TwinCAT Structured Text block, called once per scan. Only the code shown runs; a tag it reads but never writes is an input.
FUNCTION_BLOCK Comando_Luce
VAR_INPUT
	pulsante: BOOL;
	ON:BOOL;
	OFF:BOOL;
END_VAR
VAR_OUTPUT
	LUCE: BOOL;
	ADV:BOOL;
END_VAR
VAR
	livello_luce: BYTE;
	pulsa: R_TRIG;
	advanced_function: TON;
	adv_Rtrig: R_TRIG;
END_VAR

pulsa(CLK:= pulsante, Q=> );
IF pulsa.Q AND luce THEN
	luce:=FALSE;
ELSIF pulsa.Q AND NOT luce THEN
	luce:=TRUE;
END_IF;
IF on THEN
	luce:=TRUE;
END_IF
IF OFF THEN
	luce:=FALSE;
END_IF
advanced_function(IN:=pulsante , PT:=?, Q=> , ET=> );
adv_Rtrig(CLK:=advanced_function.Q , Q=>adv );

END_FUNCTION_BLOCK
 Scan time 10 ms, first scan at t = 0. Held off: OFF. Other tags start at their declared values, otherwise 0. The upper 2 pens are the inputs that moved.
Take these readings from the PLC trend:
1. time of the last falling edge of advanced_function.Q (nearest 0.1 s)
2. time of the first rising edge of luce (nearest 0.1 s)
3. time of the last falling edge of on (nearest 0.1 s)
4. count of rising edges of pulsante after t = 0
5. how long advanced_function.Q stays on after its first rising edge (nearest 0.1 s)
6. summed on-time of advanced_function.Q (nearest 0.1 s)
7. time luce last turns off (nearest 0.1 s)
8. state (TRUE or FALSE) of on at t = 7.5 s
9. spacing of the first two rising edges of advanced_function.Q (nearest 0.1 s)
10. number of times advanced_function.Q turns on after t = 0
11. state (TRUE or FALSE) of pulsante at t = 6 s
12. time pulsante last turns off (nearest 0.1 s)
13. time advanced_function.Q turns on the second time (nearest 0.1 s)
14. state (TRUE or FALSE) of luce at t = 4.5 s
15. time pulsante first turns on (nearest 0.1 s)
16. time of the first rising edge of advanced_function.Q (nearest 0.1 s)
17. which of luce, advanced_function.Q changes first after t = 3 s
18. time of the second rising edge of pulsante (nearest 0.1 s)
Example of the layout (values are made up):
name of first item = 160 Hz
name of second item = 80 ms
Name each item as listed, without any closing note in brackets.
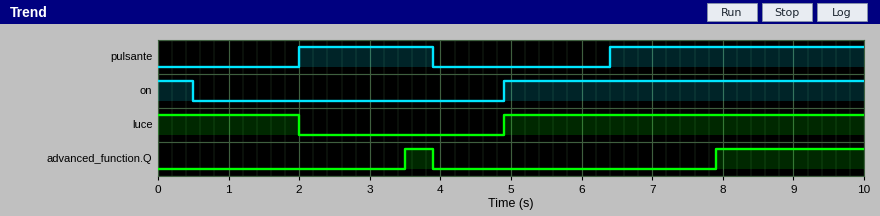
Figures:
time of the last falling edge of advanced_function.Q = 3.9 s
time of the first rising edge of luce = 4.9 s
time of the last falling edge of on = 0.5 s
count of rising edges of pulsante after t = 0 = 2
how long advanced_function.Q stays on after its first rising edge = 0.4 s
summed on-time of advanced_function.Q = 2.5 s
time luce last turns off = 2.0 s
state (TRUE or FALSE) of on at t = 7.5 s = TRUE
spacing of the first two rising edges of advanced_function.Q = 4.4 s
number of times advanced_function.Q turns on after t = 0 = 2
state (TRUE or FALSE) of pulsante at t = 6 s = FALSE
time pulsante last turns off = 3.9 s
time advanced_function.Q turns on the second time = 7.9 s
state (TRUE or FALSE) of luce at t = 4.5 s = FALSE
time pulsante first turns on = 2.0 s
time of the first rising edge of advanced_function.Q = 3.5 s
which of luce, advanced_function.Q changes first after t = 3 s = advanced_function.Q
time of the second rising edge of pulsante = 6.4 s
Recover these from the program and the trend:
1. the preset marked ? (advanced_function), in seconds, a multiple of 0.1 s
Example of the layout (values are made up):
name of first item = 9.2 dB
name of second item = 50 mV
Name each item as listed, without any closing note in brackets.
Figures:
the preset marked ? (advanced_function), in seconds, a multiple of 0.1 s = 1.5 s
